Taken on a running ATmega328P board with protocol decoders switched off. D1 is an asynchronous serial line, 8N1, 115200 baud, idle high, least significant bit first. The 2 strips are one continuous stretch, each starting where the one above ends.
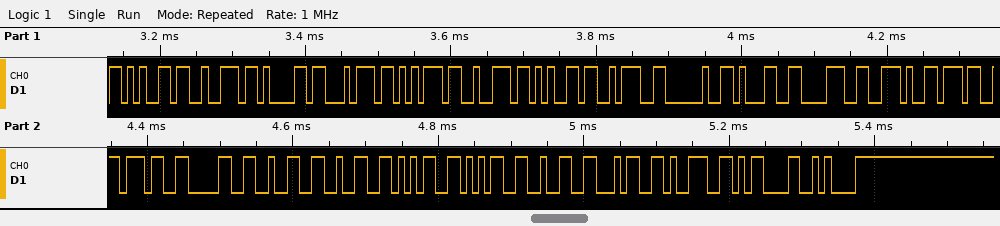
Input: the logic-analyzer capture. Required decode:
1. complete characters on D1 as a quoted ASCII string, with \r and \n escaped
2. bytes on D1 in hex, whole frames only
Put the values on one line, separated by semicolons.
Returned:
"erature: 18.7702255249\r\n"; 65 72 61 74 75 72 65 3A 20 31 38 2E 37 37 30 32 32 35 35 32 34 39 0D 0A
